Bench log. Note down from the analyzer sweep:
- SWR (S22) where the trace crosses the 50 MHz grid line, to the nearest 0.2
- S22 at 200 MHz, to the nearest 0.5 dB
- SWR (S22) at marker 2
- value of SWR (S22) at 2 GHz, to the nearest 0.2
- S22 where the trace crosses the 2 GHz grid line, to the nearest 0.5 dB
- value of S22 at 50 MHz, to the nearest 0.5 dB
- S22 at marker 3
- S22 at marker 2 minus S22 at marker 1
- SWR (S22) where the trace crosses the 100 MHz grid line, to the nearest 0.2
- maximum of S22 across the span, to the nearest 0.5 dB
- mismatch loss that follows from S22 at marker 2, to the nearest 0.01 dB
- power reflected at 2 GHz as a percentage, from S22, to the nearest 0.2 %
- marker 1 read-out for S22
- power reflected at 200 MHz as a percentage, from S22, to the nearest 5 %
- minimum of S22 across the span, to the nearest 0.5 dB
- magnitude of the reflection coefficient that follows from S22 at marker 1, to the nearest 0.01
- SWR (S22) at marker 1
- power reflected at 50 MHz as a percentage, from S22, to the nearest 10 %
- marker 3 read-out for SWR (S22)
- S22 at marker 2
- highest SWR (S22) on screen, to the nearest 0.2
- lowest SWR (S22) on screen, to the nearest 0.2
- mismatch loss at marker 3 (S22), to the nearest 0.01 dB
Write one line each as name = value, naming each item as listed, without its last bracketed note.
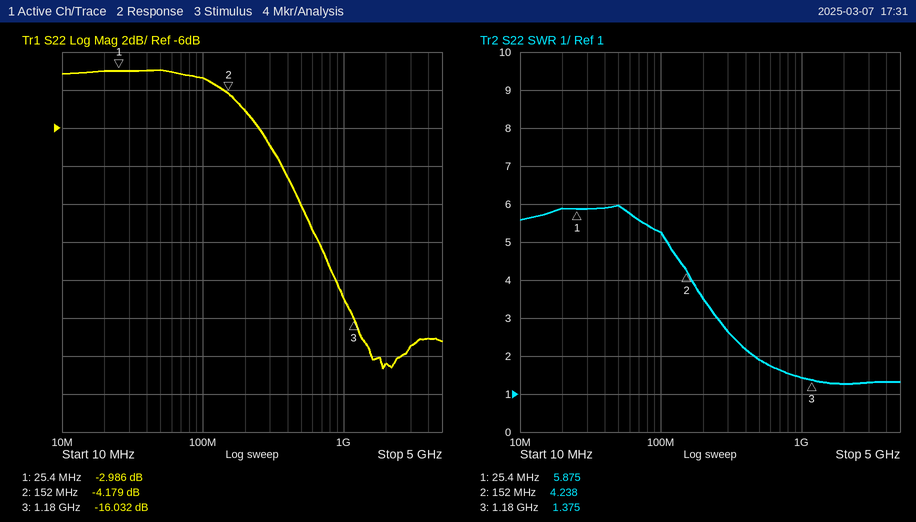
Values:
SWR (S22) where the trace crosses the 50 MHz grid line, to the nearest 0.2 = 6.0
S22 at 200 MHz, to the nearest 0.5 dB = -5.0 dB
SWR (S22) at marker 2 = 4.238
value of SWR (S22) at 2 GHz, to the nearest 0.2 = 1.2
S22 where the trace crosses the 2 GHz grid line, to the nearest 0.5 dB = -18.5 dB
value of S22 at 50 MHz, to the nearest 0.5 dB = -3.0 dB
S22 at marker 3 = -16.032 dB
S22 at marker 2 minus S22 at marker 1 = -1.193 dB
SWR (S22) where the trace crosses the 100 MHz grid line, to the nearest 0.2 = 5.2
maximum of S22 across the span, to the nearest 0.5 dB = -3.0 dB
mismatch loss that follows from S22 at marker 2, to the nearest 0.01 dB = 2.09 dB
power reflected at 2 GHz as a percentage, from S22, to the nearest 0.2 % = 1.4 %
marker 1 read-out for S22 = -2.986 dB
power reflected at 200 MHz as a percentage, from S22, to the nearest 5 % = 30 %
minimum of S22 across the span, to the nearest 0.5 dB = -18.5 dB
magnitude of the reflection coefficient that follows from S22 at marker 1, to the nearest 0.01 = 0.71
SWR (S22) at marker 1 = 5.875
power reflected at 50 MHz as a percentage, from S22, to the nearest 10 % = 50 %
marker 3 read-out for SWR = 1.375
S22 at marker 2 = -4.179 dB
highest SWR (S22) on screen, to the nearest 0.2 = 6.0
lowest SWR (S22) on screen, to the nearest 0.2 = 1.2
mismatch loss at marker 3 (S22), to the nearest 0.01 dB = 0.11 dB
